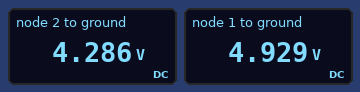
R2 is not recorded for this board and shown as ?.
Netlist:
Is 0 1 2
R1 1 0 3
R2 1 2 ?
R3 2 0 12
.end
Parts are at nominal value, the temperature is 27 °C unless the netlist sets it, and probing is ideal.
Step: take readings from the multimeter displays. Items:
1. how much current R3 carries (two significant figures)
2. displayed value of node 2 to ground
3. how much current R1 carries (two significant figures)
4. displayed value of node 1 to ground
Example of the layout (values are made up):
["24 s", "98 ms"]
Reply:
["360 mA", "4.286 V", "1.6 A", "4.929 V"]
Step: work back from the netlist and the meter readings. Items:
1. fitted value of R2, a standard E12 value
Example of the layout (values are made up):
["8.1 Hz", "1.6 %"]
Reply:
["1.8 Ω"]
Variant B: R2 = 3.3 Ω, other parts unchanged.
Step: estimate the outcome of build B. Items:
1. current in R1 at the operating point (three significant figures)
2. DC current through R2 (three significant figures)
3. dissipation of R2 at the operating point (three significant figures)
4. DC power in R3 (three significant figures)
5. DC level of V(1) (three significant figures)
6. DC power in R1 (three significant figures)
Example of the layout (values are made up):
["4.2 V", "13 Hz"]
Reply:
["1.67 A", "328 mA", "355 mW", "1.29 W", "5.02 V", "8.39 W"]
